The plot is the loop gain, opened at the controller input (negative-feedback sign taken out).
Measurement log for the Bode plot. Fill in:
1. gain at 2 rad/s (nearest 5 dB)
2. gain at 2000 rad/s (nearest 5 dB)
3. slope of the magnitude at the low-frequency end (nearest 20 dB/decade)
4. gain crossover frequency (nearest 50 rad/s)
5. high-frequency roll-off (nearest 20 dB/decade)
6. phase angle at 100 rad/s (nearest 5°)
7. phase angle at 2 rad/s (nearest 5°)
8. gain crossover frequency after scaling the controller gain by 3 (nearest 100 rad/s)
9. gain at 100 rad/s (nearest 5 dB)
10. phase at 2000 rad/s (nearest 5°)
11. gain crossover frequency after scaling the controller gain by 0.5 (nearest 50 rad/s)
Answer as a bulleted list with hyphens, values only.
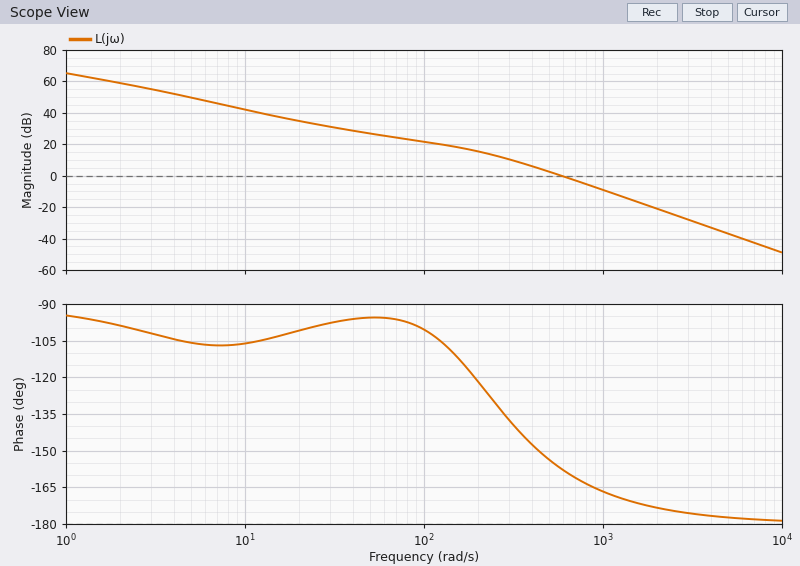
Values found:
- 60 dB
- -20 dB
- -20 dB/decade
- 600 rad/s
- -40 dB/decade
- -100°
- -100°
- 1000 rad/s
- 20 dB
- -175°
- 400 rad/s
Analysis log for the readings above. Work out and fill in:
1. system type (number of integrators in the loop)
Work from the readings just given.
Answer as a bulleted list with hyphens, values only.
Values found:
- 1
